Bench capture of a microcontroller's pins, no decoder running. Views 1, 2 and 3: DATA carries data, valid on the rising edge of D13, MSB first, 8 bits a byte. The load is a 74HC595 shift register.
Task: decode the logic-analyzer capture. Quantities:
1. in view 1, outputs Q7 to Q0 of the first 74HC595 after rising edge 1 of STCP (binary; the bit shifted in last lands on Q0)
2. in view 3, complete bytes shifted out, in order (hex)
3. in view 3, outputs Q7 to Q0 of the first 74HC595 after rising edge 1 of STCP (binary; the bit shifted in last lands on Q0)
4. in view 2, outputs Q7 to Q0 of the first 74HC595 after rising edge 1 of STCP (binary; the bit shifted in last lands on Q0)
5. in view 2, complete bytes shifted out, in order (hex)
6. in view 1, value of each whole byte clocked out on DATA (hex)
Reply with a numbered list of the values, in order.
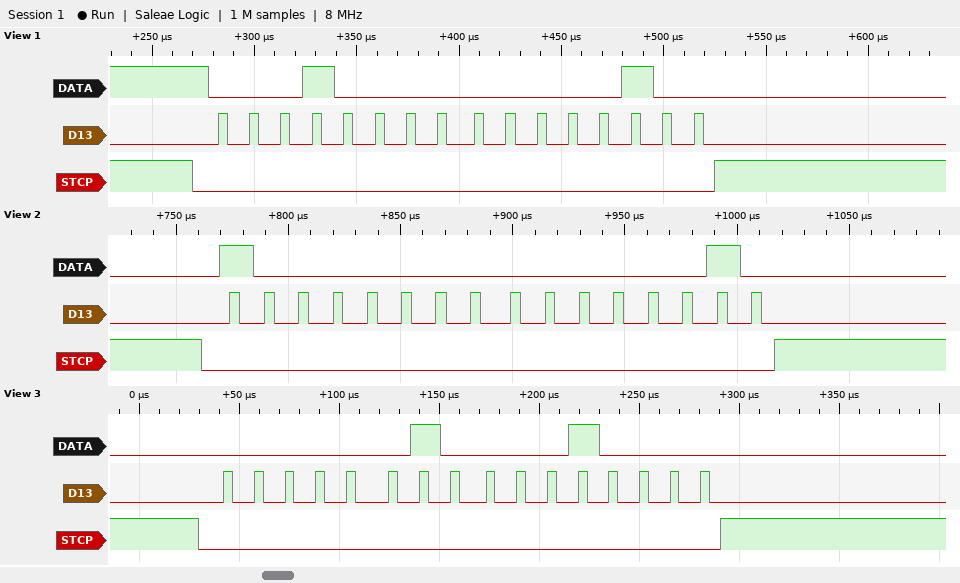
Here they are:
1. 00000100
2. 02 10
3. 00010000
4. 00000010
5. 80 02
6. 0x10 0x04
